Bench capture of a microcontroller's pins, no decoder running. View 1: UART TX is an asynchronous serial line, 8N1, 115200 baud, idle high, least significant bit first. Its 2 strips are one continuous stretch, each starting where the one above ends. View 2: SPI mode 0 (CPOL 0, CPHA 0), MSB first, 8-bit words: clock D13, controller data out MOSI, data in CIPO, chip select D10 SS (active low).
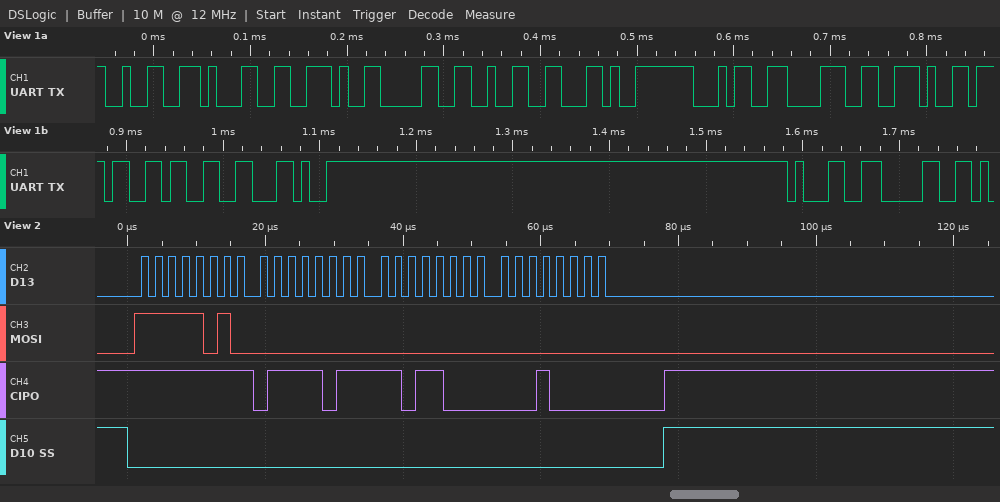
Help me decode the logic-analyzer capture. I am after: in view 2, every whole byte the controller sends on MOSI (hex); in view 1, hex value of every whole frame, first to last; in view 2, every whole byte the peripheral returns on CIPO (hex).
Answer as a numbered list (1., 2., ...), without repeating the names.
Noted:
1. FA 00 00 00
2. 0x32 0x31 0x2E 0x30 0x32 0x2C 0x34 0x38 0x2E 0x37 0x33 0x2C 0x31 0x30
3. FF 7B D8 10
